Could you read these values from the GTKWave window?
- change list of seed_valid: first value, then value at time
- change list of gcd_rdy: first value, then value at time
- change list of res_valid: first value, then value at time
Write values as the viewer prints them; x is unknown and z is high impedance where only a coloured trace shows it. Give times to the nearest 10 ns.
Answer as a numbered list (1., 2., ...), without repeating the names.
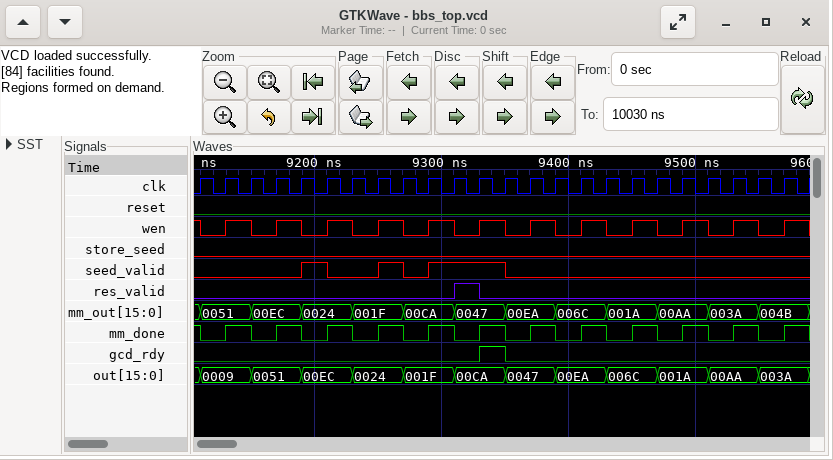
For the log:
1. 0, 1 at 9190 ns, 0 at 9210 ns, 1 at 9250 ns, 0 at 9270 ns, 1 at 9290 ns, 0 at 9350 ns
2. 0, 1 at 9330 ns, 0 at 9350 ns
3. 0, 1 at 9310 ns, 0 at 9330 ns
